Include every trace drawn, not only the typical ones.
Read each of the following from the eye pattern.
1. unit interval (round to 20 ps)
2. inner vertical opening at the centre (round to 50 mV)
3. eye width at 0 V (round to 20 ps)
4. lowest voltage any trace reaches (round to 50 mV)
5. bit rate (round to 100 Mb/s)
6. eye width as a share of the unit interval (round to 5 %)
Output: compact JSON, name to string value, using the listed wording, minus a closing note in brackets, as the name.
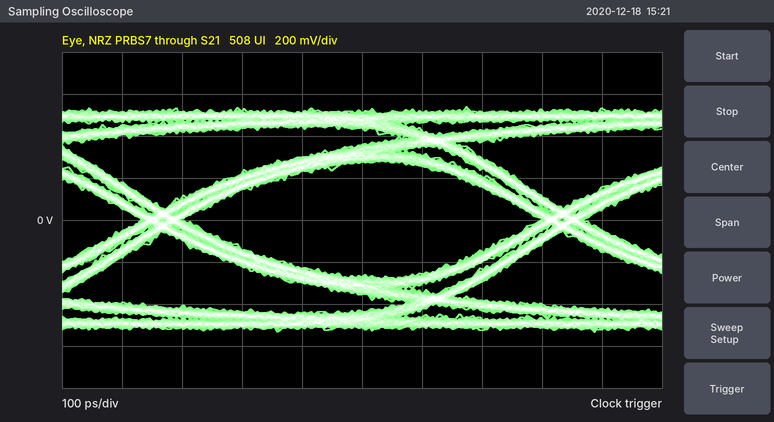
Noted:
{"unit interval": "660 ps", "inner vertical opening at the centre": "550 mV", "eye width at 0 V": "600 ps", "lowest voltage any trace reaches": "-550 mV", "bit rate": "1.5 Gb/s", "eye width as a share of the unit interval": "90 %"}
